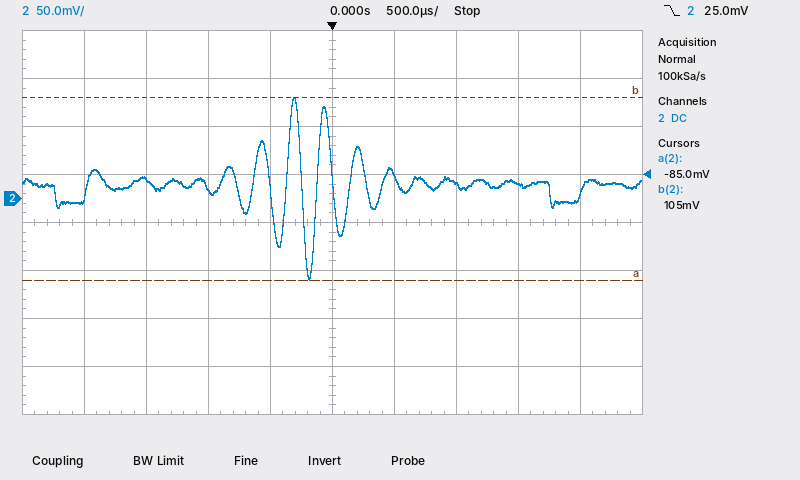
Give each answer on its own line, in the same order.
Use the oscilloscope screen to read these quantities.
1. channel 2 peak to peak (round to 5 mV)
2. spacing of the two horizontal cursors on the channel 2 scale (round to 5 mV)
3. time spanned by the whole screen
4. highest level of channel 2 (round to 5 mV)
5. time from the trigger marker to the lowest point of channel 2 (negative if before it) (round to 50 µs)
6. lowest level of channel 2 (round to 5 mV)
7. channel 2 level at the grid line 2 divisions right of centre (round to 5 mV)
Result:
190 mV
190 mV
5 ms
105 mV
-200 µs
-85 mV
15 mV
